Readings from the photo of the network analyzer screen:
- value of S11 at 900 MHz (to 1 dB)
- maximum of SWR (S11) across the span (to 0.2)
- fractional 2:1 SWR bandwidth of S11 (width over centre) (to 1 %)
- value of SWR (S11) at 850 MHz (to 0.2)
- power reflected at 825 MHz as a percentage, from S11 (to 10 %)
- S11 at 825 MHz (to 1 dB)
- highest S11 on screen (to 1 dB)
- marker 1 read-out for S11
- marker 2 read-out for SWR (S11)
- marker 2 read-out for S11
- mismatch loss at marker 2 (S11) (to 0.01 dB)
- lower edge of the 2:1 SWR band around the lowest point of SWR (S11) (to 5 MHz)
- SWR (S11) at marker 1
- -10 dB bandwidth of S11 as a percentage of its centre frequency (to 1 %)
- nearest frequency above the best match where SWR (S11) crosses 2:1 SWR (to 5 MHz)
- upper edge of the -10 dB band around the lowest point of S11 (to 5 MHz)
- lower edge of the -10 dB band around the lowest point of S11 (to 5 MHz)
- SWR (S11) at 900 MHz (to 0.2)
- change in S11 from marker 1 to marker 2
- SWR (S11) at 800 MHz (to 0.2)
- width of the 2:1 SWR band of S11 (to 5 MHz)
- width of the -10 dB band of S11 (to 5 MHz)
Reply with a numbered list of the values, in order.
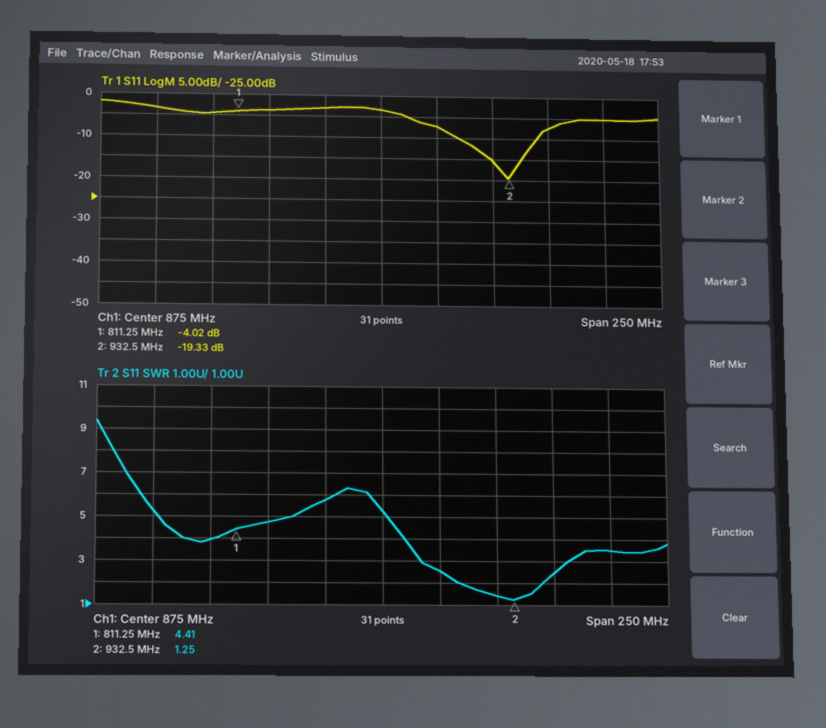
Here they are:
1. -7 dB
2. 9.4
3. 4 %
4. 5.8
5. 40 %
6. -4 dB
7. -2 dB
8. -4.02 dB
9. 1.25
10. -19.33 dB
11. 0.05 dB
12. 910 MHz
13. 4.41
14. 4 %
15. 945 MHz
16. 945 MHz
17. 910 MHz
18. 2.6
19. -15.31 dB
20. 4.0
21. 35 MHz
22. 35 MHz
